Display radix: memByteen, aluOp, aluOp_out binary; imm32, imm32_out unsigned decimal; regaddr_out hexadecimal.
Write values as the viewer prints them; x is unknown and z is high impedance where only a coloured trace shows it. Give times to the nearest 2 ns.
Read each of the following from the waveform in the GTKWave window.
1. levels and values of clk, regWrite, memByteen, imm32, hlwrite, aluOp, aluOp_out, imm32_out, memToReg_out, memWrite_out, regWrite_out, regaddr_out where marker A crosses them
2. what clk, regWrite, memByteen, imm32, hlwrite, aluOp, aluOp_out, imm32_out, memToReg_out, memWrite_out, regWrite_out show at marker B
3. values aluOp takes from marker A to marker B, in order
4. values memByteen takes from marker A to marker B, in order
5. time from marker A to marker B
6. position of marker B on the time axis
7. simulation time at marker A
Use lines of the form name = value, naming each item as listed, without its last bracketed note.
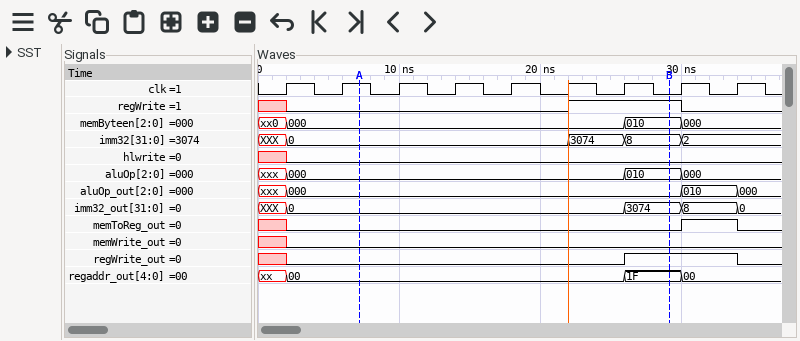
levels and values of clk, regWrite, memByteen, imm32, hlwrite, aluOp, aluOp_out, imm32_out, memToReg_out, memWrite_out, regWrite_out, regaddr_out where marker A crosses them = clk=1, regWrite=0, memByteen=000, imm32=0, hlwrite=0, aluOp=000, aluOp_out=000, imm32_out=0, memToReg_out=0, memWrite_out=0, regWrite_out=0, regaddr_out=00
what clk, regWrite, memByteen, imm32, hlwrite, aluOp, aluOp_out, imm32_out, memToReg_out, memWrite_out, regWrite_out show at marker B = clk=0, regWrite=1, memByteen=010, imm32=8, hlwrite=0, aluOp=010, aluOp_out=000, imm32_out=3074, memToReg_out=0, memWrite_out=0, regWrite_out=1
values aluOp takes from marker A to marker B, in order = 000, 010
values memByteen takes from marker A to marker B, in order = 000, 010
time from marker A to marker B = 22 ns
position of marker B on the time axis = 30 ns
simulation time at marker A = 8 ns
